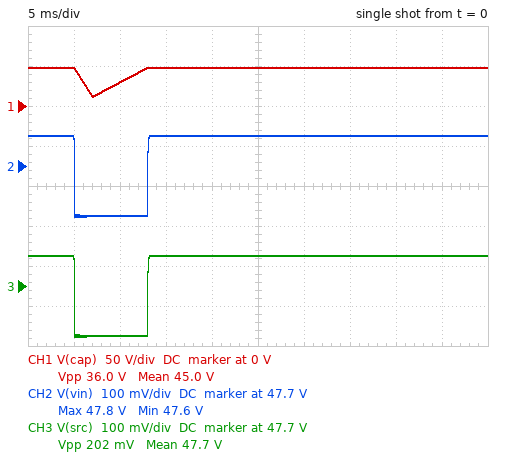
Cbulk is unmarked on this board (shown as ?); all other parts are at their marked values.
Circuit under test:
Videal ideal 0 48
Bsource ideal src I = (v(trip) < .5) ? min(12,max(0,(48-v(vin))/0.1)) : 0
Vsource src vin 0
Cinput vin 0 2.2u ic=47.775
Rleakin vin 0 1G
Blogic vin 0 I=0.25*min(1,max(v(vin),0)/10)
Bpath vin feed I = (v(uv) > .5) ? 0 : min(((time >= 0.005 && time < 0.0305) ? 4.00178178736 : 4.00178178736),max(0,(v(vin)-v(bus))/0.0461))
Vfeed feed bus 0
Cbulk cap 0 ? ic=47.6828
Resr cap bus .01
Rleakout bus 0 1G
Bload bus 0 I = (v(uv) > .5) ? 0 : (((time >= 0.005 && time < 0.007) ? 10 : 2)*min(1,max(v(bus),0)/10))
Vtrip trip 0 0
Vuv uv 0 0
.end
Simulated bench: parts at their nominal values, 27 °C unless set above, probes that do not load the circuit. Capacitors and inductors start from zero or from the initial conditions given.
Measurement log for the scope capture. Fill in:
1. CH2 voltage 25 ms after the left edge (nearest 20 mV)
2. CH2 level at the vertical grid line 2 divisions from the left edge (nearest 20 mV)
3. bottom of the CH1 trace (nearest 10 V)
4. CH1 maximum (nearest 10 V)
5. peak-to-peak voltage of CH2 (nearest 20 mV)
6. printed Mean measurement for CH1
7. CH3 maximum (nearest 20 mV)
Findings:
47.78 V
47.58 V
10 V
50 V
200 mV
45.0 V
47.78 V
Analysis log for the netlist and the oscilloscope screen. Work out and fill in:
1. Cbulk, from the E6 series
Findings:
330 µF
